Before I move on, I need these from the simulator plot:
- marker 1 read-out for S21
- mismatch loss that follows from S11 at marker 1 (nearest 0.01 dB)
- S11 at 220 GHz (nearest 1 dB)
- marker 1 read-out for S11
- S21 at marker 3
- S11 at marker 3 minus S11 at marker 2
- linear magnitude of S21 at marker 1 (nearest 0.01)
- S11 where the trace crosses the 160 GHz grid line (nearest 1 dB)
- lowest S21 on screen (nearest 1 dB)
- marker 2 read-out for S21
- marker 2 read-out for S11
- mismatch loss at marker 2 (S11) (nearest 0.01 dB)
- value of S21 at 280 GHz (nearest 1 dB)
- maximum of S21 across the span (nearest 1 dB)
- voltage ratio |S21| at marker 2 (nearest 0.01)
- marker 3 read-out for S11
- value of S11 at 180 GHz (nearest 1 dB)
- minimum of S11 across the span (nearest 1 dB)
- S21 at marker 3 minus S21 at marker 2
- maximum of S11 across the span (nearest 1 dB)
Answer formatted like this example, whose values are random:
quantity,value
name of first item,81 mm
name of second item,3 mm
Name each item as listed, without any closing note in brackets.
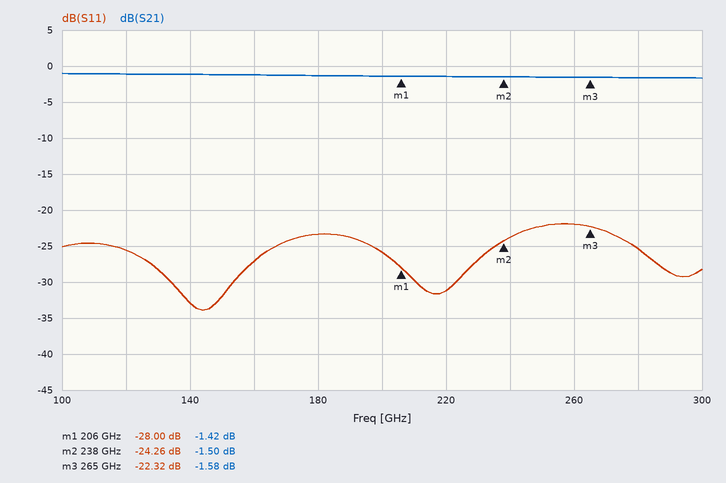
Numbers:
quantity,value
marker 1 read-out for S21,-1.42 dB
mismatch loss that follows from S11 at marker 1,0.01 dB
S11 at 220 GHz,-31 dB
marker 1 read-out for S11,-28.00 dB
S21 at marker 3,-1.58 dB
S11 at marker 3 minus S11 at marker 2,1.94 dB
linear magnitude of S21 at marker 1,0.85
S11 where the trace crosses the 160 GHz grid line,-27 dB
lowest S21 on screen,-2 dB
marker 2 read-out for S21,-1.50 dB
marker 2 read-out for S11,-24.26 dB
mismatch loss at marker 2 (S11),0.02 dB
value of S21 at 280 GHz,-2 dB
maximum of S21 across the span,-1 dB
voltage ratio |S21| at marker 2,0.84
marker 3 read-out for S11,-22.32 dB
value of S11 at 180 GHz,-23 dB
minimum of S11 across the span,-34 dB
S21 at marker 3 minus S21 at marker 2,-0.08 dB
maximum of S11 across the span,-22 dB
